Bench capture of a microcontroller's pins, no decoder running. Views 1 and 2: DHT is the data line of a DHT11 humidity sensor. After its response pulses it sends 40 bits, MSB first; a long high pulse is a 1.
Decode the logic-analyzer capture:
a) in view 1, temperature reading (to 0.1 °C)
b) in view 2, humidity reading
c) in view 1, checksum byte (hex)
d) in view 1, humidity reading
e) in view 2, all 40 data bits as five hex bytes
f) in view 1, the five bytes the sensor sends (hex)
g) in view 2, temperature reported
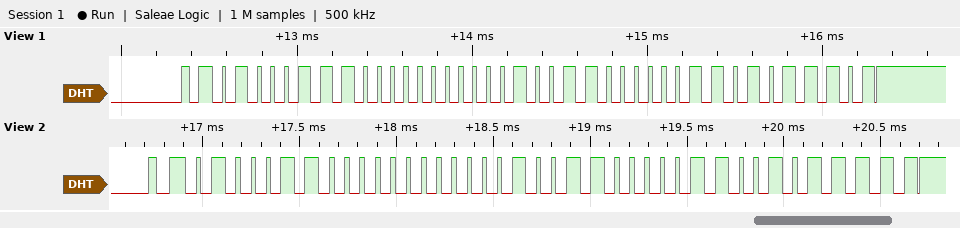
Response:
19.3 °C
70 %
0x5D
71 %
46 00 13 06 5F
47 00 13 03 5D
19.6 °C
